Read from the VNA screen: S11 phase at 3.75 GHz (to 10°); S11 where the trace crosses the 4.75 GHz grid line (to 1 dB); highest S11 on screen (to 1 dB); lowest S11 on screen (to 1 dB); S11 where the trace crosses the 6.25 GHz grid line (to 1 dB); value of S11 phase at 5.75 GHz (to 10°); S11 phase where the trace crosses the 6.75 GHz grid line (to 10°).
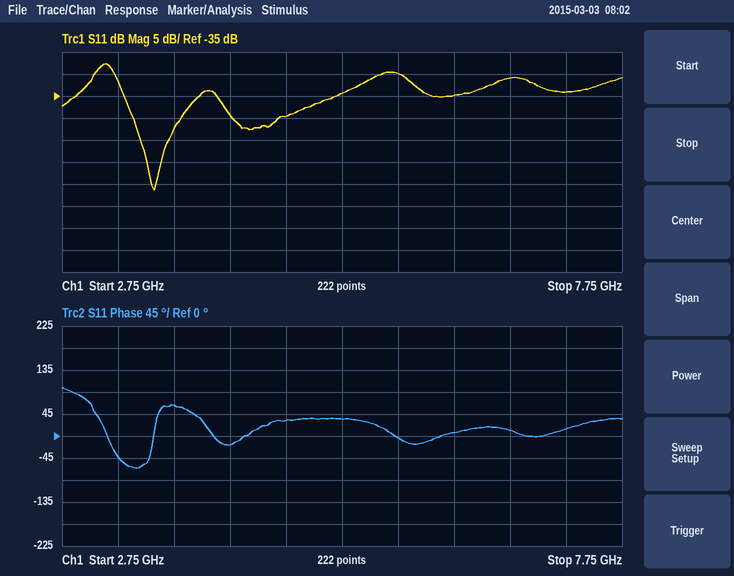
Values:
60°
-40 dB
-28 dB
-56 dB
-35 dB
0°
10°
